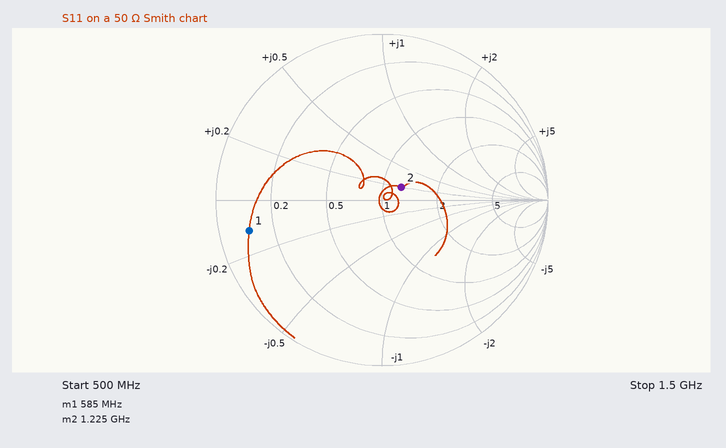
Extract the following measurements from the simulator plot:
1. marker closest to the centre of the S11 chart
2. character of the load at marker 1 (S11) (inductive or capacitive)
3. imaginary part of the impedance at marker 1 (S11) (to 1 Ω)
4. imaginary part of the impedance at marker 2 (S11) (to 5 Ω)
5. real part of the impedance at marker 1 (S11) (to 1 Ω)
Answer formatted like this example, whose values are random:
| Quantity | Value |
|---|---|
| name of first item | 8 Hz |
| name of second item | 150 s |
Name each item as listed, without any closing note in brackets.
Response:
| Quantity | Value |
|---|---|
| marker closest to the centre of the S11 chart | marker 2 |
| character of the load at marker 1 (S11) | capacitive |
| imaginary part of the impedance at marker 1 (S11) | -6 Ω |
| imaginary part of the impedance at marker 2 (S11) | +10 Ω |
| real part of the impedance at marker 1 (S11) | 5 Ω |
